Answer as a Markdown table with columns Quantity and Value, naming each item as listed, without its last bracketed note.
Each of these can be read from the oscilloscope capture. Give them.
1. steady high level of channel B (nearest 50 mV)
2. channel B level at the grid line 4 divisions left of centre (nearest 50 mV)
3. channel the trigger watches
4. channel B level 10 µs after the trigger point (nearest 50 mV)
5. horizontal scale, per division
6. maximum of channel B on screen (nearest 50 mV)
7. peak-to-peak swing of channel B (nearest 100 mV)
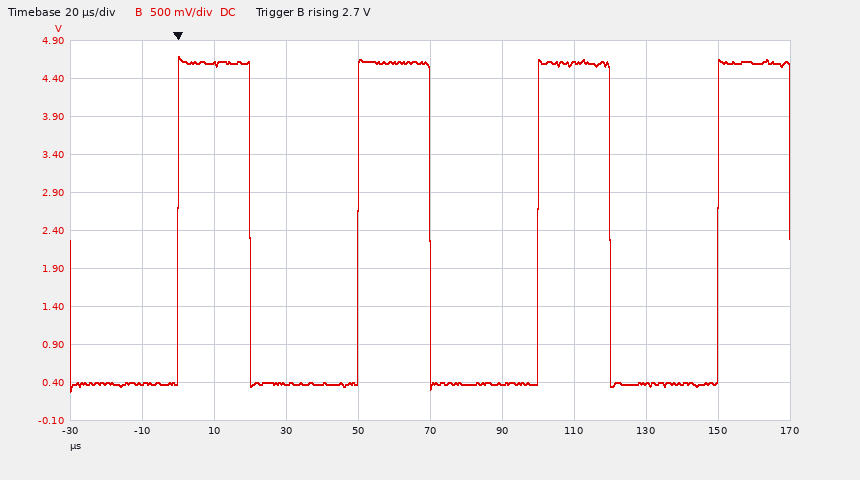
| Quantity | Value |
|---|---|
| steady high level of channel B | 4.60 V |
| channel B level at the grid line 4 divisions left of centre | 400 mV |
| channel the trigger watches | channel B |
| channel B level 10 µs after the trigger point | 4.60 V |
| horizontal scale, per division | 20 µs |
| maximum of channel B on screen | 4.70 V |
| peak-to-peak swing of channel B | 4.40 V |
